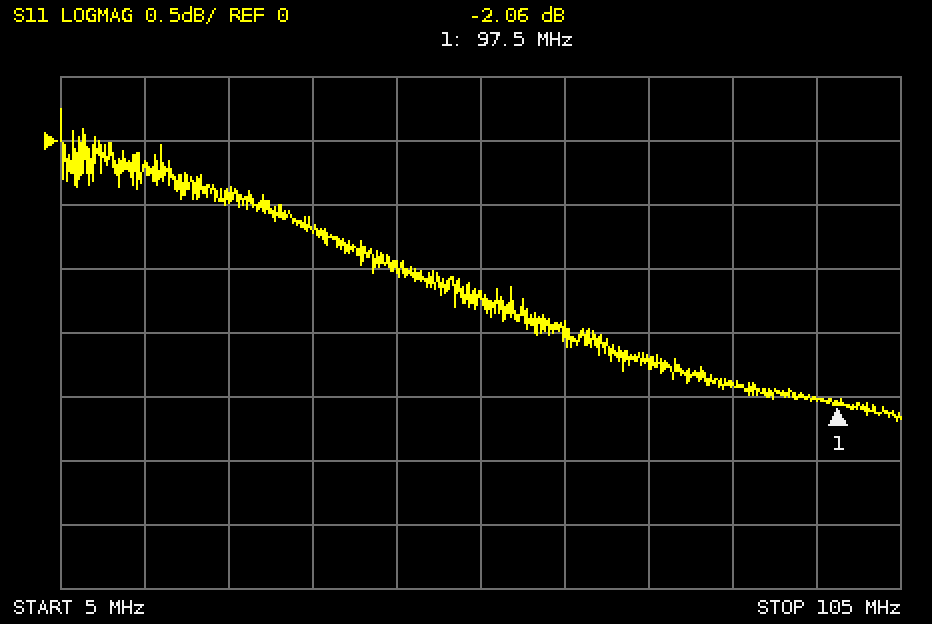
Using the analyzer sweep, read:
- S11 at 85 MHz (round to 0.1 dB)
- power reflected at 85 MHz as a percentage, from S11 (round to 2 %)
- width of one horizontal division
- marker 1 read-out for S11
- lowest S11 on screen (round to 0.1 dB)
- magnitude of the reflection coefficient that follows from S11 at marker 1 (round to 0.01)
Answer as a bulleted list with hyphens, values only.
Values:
- -1.9 dB
- 64 %
- 10 MHz
- -2.06 dB
- -2.2 dB
- 0.79
